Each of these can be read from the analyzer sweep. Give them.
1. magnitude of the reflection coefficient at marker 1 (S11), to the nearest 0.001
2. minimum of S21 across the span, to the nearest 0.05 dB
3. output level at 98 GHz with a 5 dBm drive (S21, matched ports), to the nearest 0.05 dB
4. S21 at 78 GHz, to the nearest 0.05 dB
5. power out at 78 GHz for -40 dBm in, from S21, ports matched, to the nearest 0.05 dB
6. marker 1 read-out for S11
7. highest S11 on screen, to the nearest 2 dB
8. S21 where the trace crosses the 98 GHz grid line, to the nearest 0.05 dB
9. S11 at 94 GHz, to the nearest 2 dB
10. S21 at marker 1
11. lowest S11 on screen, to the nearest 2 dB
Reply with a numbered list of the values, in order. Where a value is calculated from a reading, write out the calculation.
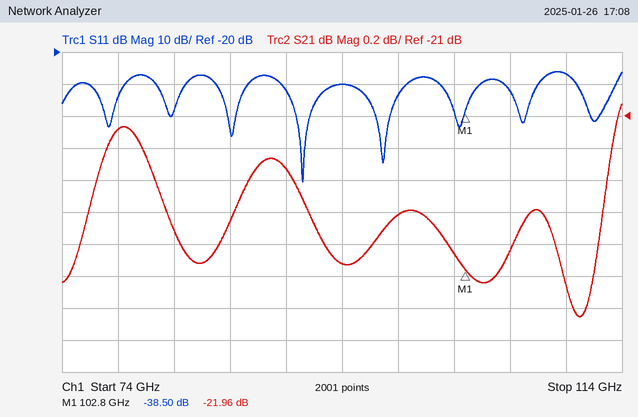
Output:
1. 10^(-38.5/20) ≈ 0.012
2. -22.25 dB
3. 5 dBm + (-21.60 dB) = -16.60 dBm
4. -21.10 dB
5. -40 dBm + (-21.10 dB) = -61.10 dBm
6. -38.50 dB
7. -26 dB
8. -21.60 dB
9. -30 dB
10. -21.96 dB
11. -60 dB
